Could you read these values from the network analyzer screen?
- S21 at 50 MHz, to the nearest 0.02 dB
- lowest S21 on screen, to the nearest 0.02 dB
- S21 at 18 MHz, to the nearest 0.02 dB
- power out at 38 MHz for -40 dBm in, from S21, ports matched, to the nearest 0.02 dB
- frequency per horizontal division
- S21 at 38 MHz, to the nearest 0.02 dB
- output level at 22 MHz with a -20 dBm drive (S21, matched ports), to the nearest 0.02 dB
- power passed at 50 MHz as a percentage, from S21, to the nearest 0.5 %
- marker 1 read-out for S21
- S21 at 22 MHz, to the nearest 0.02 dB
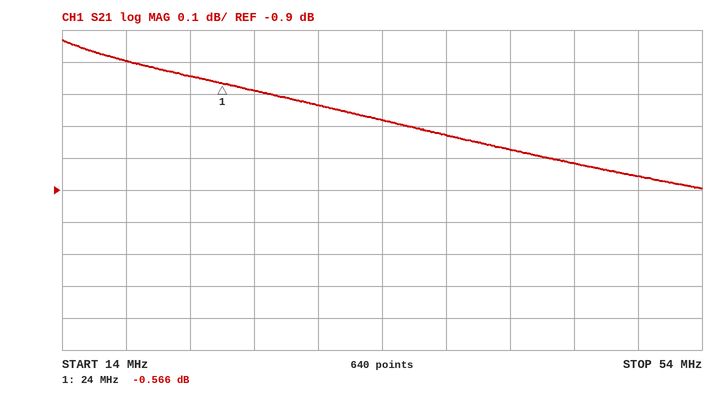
-0.86 dB
-0.90 dB
-0.50 dB
-40.72 dBm
4 MHz
-0.72 dB
-20.54 dBm
82.0 %
-0.566 dB
-0.54 dB
